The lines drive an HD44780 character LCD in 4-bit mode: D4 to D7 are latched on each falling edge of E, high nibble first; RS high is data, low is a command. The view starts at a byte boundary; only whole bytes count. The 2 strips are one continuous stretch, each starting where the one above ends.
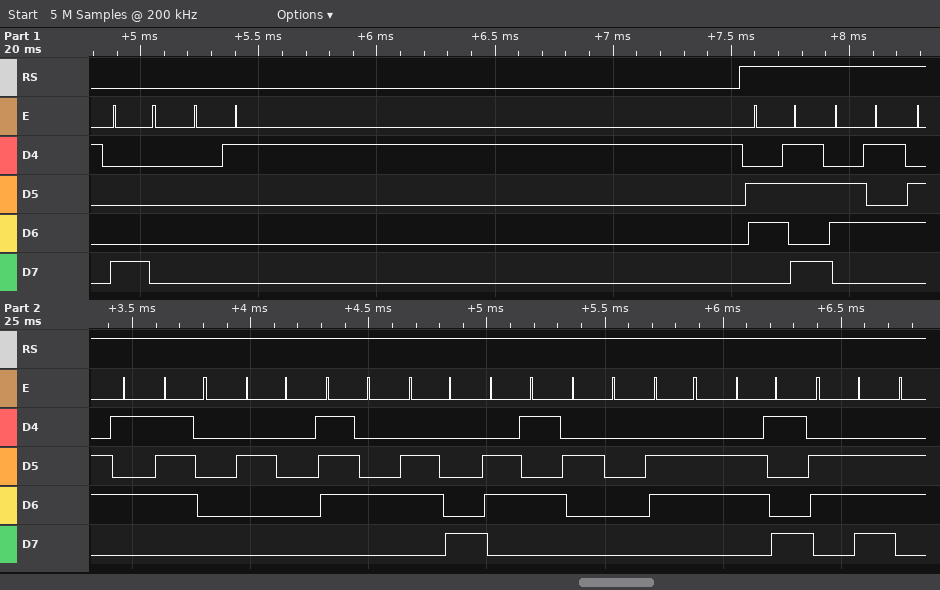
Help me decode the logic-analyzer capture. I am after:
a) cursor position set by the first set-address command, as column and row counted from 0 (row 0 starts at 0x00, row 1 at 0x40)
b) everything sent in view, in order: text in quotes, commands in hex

column 0, row 0
0x80 0x01 "keep the fin"
